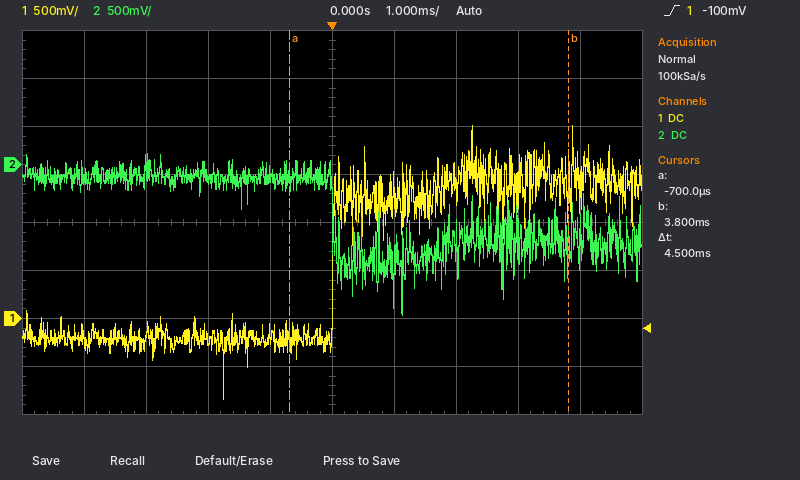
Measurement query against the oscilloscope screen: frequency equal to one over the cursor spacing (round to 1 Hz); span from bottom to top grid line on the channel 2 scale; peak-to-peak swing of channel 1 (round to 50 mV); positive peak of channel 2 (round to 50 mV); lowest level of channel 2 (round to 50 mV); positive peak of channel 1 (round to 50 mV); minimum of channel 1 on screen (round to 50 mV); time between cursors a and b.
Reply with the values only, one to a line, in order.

222 Hz
4 V
2.85 V
100 mV
-1.55 V
2.00 V
-850 mV
4.5 ms
